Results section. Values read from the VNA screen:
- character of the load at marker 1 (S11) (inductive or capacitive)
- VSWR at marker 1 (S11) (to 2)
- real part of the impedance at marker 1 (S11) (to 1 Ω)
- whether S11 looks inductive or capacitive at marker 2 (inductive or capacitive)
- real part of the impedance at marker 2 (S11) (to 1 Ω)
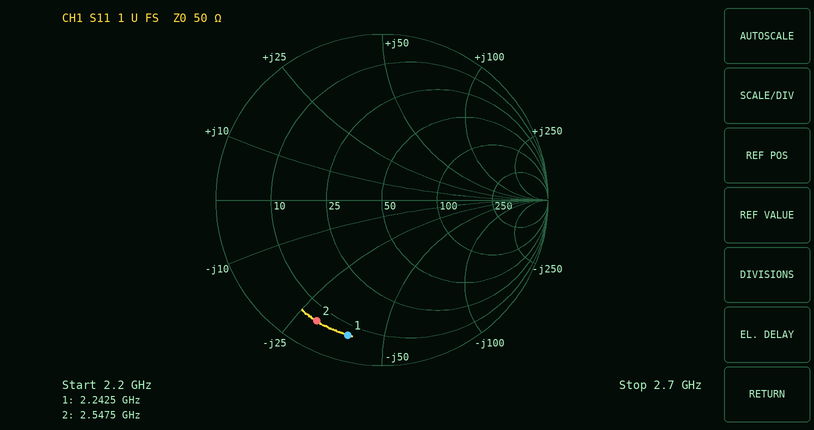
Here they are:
capacitive
12
7 Ω
capacitive
6 Ω
